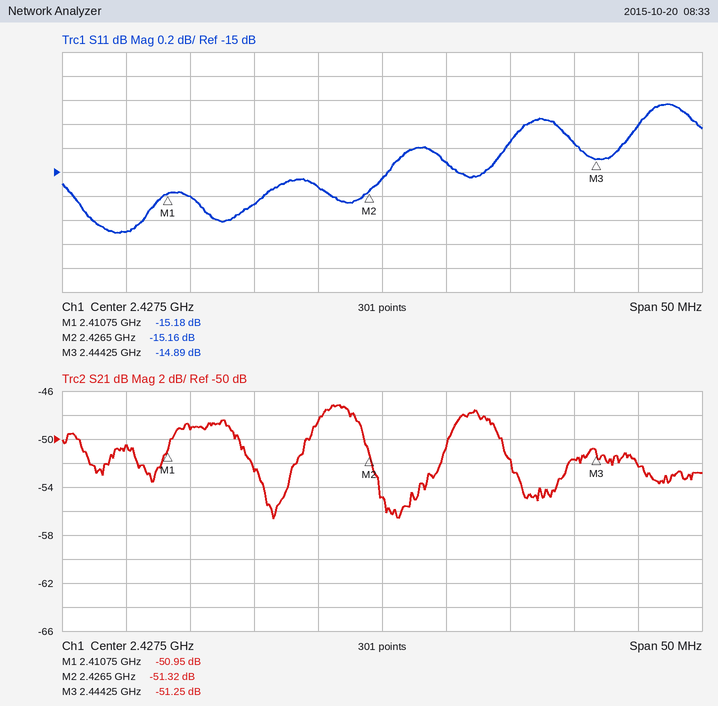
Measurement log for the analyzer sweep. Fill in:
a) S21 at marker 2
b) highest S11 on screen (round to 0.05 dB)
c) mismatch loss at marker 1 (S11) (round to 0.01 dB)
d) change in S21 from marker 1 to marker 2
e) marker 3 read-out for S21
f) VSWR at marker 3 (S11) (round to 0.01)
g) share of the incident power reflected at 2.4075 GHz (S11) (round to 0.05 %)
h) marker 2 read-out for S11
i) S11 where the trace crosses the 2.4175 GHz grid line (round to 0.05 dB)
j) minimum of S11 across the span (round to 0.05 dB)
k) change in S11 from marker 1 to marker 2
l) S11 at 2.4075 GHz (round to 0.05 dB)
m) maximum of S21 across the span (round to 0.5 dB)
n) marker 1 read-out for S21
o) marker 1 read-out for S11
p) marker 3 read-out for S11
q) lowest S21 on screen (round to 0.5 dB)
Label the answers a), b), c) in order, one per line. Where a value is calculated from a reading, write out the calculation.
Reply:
a) -51.32 dB
b) -14.45 dB
c) −10 log10(1 − 10^(-15.18/10)) ≈ 0.13 dB
d) -51.32 − (-50.95) = -0.37 dB
e) -51.25 dB
f) (1 + 0.1801)/(1 − 0.1801) ≈ 1.44
g) 10^(-15.5/10) ≈ 2.82 %, so 2.80 % to the nearest 0.05 %
h) -15.16 dB
i) -15.25 dB
j) -15.50 dB
k) -15.16 − (-15.18) = 0.02 dB
l) -15.50 dB
m) -47.0 dB
n) -50.95 dB
o) -15.18 dB
p) -14.89 dB
q) -56.5 dB
